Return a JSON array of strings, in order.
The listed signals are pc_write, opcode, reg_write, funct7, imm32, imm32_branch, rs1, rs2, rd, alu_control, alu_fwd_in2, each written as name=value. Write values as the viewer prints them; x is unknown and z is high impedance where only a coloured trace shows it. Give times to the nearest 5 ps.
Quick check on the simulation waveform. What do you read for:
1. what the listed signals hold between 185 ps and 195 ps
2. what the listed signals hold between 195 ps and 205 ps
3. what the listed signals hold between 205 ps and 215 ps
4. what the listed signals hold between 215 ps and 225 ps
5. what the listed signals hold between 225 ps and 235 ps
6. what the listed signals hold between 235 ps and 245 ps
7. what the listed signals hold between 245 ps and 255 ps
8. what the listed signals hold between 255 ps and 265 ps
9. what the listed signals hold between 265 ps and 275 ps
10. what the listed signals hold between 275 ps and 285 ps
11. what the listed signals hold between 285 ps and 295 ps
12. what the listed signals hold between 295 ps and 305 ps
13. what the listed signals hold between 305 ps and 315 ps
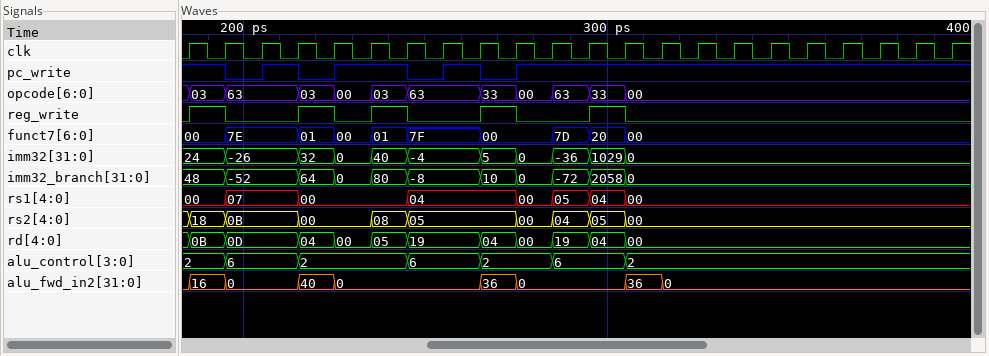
["pc_write=1, opcode=03, reg_write=1, funct7=00, imm32=24, imm32_branch=48, rs1=00, rs2=18, rd=0B, alu_control=2, alu_fwd_in2=16", "pc_write=0, opcode=63, reg_write=0, funct7=7E, imm32=-26, imm32_branch=-52, rs1=07, rs2=0B, rd=0D, alu_control=6, alu_fwd_in2=0", "pc_write=1, opcode=63, reg_write=0, funct7=7E, imm32=-26, imm32_branch=-52, rs1=07, rs2=0B, rd=0D, alu_control=6, alu_fwd_in2=0", "pc_write=0, opcode=03, reg_write=1, funct7=01, imm32=32, imm32_branch=64, rs1=00, rs2=00, rd=04, alu_control=2, alu_fwd_in2=40", "pc_write=1, opcode=00, reg_write=0, funct7=00, imm32=0, imm32_branch=0, rs1=00, rs2=00, rd=00, alu_control=2, alu_fwd_in2=0", "pc_write=1, opcode=03, reg_write=1, funct7=01, imm32=40, imm32_branch=80, rs1=00, rs2=08, rd=05, alu_control=2, alu_fwd_in2=0", "pc_write=0, opcode=63, reg_write=0, funct7=7F, imm32=-4, imm32_branch=-8, rs1=04, rs2=05, rd=19, alu_control=6, alu_fwd_in2=0", "pc_write=1, opcode=63, reg_write=0, funct7=7F, imm32=-4, imm32_branch=-8, rs1=04, rs2=05, rd=19, alu_control=6, alu_fwd_in2=0", "pc_write=0, opcode=33, reg_write=1, funct7=00, imm32=5, imm32_branch=10, rs1=04, rs2=05, rd=04, alu_control=2, alu_fwd_in2=36", "pc_write=1, opcode=00, reg_write=0, funct7=00, imm32=0, imm32_branch=0, rs1=00, rs2=00, rd=00, alu_control=2, alu_fwd_in2=0", "pc_write=1, opcode=63, reg_write=0, funct7=7D, imm32=-36, imm32_branch=-72, rs1=05, rs2=04, rd=19, alu_control=6, alu_fwd_in2=0", "pc_write=1, opcode=33, reg_write=1, funct7=20, imm32=1029, imm32_branch=2058, rs1=04, rs2=05, rd=04, alu_control=6, alu_fwd_in2=0", "pc_write=1, opcode=00, reg_write=0, funct7=00, imm32=0, imm32_branch=0, rs1=00, rs2=00, rd=00, alu_control=2, alu_fwd_in2=36"]
